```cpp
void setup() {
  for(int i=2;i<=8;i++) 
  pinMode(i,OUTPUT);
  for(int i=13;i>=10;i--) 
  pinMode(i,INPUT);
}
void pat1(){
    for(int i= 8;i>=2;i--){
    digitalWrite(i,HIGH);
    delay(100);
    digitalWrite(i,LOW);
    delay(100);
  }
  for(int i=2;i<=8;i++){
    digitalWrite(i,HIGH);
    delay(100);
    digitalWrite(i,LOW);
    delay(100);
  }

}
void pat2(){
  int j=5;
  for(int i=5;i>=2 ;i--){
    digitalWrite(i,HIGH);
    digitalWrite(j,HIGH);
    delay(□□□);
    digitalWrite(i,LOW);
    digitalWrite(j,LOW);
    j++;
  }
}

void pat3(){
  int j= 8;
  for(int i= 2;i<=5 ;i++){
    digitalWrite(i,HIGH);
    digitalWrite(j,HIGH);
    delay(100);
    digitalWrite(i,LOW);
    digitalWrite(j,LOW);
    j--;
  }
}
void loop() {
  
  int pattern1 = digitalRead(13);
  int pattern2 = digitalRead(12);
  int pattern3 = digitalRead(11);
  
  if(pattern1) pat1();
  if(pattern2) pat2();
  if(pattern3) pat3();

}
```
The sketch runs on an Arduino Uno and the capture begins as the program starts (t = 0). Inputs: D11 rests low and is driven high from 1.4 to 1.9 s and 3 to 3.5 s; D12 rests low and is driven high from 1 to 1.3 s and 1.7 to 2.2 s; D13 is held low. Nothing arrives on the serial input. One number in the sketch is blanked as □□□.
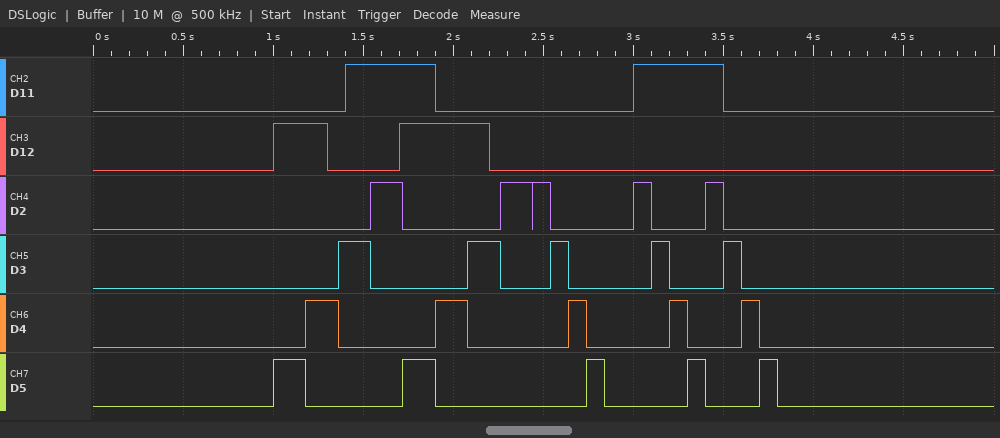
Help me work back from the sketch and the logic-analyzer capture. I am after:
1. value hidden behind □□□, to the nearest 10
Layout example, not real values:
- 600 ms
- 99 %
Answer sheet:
- 180
